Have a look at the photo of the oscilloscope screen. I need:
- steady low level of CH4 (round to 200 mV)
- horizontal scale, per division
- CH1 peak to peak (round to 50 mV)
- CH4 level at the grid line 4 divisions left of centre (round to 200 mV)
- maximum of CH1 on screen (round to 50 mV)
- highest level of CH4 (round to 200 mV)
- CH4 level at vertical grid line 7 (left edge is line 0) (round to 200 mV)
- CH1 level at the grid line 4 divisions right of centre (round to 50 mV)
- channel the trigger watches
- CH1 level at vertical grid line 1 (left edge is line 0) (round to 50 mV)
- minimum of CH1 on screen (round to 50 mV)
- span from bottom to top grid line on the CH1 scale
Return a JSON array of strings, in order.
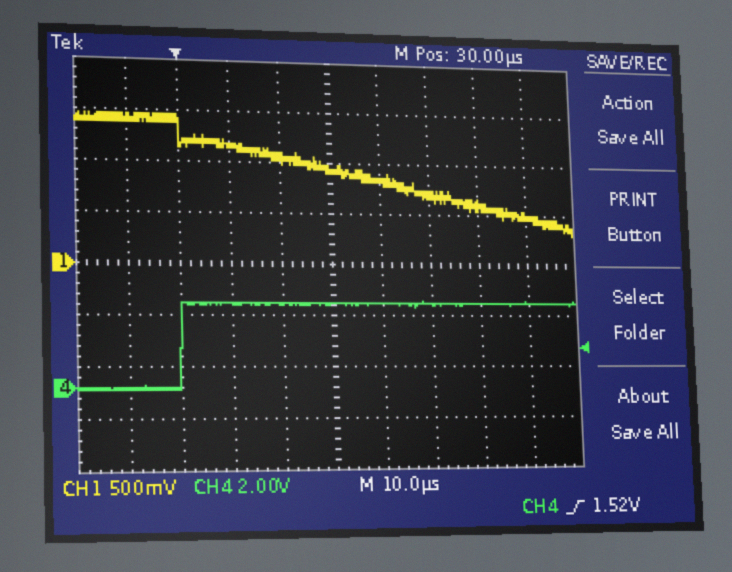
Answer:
["0.0 V", "10 µs", "1.15 V", "0.0 V", "1.45 V", "3.4 V", "3.2 V", "500 mV", "CH4", "1.40 V", "300 mV", "4 V"]
